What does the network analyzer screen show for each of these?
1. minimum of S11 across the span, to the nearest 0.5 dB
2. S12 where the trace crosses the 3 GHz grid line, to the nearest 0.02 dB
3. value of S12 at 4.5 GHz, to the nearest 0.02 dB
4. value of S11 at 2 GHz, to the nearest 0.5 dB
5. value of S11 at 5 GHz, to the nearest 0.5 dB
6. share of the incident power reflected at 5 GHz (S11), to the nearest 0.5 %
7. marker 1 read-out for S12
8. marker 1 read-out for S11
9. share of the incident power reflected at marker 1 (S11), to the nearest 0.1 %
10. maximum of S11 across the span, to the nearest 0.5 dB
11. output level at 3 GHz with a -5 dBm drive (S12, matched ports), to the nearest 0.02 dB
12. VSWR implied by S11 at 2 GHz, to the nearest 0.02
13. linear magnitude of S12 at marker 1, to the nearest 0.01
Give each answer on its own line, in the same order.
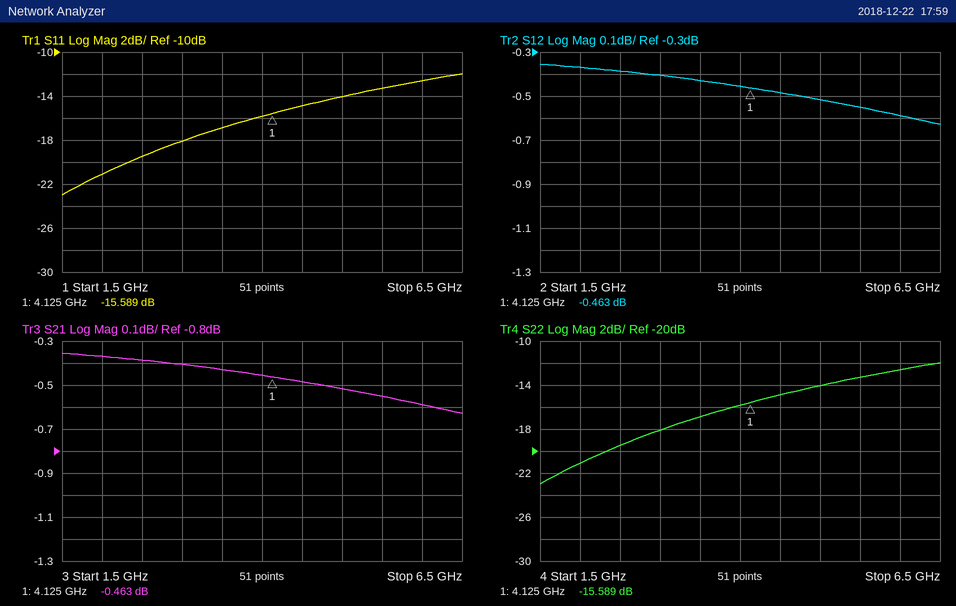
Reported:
-23.0 dB
-0.40 dB
-0.48 dB
-21.0 dB
-14.0 dB
4.0 %
-0.463 dB
-15.589 dB
2.8 %
-12.0 dB
-5.40 dBm
1.20
0.95
